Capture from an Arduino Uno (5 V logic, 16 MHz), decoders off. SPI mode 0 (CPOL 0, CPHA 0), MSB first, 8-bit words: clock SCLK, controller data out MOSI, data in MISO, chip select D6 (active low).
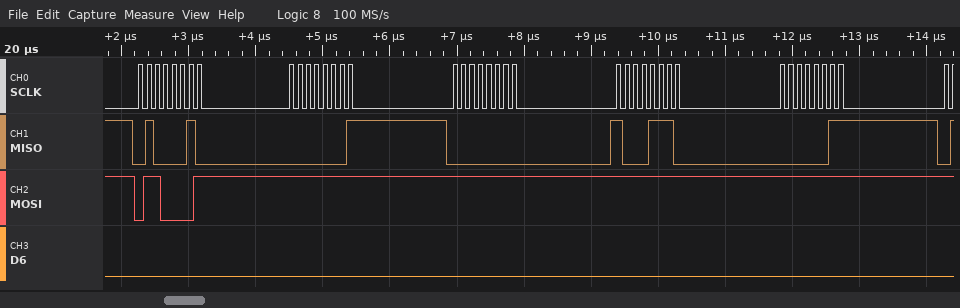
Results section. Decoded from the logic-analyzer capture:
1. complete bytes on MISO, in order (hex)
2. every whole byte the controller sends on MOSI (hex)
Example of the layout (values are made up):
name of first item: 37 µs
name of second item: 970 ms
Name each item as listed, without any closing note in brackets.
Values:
complete bytes on MISO, in order: 42 01 00 8E 03
every whole byte the controller sends on MOSI: 61 FF FF FF FF
